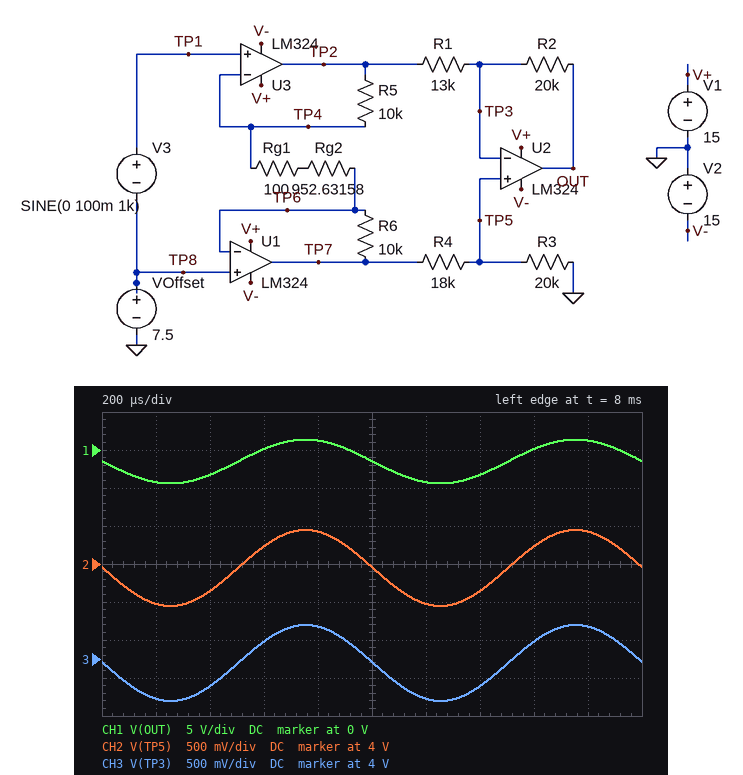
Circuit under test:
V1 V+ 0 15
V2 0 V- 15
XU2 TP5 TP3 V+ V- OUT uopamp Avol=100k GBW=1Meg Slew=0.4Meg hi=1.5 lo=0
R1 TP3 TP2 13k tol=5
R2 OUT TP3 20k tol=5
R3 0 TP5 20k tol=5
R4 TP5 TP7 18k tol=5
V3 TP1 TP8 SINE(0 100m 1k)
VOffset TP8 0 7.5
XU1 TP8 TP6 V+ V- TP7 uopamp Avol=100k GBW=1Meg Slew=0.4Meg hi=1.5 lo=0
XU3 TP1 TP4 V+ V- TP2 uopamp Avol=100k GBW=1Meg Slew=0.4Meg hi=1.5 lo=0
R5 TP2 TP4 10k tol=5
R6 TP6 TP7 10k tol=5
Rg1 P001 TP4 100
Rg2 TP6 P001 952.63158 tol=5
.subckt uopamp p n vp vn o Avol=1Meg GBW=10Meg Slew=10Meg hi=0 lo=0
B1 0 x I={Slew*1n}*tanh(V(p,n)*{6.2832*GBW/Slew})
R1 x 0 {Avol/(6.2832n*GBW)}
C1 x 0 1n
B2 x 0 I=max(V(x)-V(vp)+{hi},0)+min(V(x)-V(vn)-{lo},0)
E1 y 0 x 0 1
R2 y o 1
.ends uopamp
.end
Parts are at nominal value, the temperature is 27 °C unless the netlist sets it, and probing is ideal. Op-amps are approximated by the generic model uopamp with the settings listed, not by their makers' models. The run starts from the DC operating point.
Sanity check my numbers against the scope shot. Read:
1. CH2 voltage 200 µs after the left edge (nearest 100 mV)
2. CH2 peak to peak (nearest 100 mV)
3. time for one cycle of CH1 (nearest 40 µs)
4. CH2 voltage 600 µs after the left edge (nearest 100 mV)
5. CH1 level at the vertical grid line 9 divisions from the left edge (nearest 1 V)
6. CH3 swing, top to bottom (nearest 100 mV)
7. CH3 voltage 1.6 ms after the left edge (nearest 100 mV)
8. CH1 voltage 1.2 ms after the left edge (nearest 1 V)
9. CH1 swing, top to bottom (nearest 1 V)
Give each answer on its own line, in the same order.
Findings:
3.5 V
1.0 V
1.00 ms
4.2 V
1 V
1.0 V
4.2 V
-4 V
6 V
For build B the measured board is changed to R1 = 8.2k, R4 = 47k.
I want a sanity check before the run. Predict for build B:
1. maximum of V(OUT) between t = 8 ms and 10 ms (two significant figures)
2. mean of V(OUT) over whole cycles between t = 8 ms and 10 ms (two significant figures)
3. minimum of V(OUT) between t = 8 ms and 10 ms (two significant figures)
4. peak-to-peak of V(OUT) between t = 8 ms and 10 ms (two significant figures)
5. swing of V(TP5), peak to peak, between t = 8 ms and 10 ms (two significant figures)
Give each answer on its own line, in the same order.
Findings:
-7.1 V
-11 V
-14 V
7.1 V
570 mV
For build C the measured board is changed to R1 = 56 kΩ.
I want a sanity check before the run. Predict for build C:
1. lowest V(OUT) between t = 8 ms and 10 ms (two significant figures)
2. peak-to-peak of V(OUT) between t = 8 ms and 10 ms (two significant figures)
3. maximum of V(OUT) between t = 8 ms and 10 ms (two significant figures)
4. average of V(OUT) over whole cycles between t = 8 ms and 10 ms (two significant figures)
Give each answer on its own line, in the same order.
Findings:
1.6 V
2.1 V
3.7 V
2.7 V
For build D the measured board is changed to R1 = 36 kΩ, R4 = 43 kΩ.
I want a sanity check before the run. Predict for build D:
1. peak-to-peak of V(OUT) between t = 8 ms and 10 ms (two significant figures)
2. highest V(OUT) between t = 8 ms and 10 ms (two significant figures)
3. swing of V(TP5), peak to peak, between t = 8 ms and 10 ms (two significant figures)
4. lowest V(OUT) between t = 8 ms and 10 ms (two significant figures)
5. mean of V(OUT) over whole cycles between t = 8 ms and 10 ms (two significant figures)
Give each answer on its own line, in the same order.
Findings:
2.1 V
590 mV
600 mV
-1.5 V
-460 mV
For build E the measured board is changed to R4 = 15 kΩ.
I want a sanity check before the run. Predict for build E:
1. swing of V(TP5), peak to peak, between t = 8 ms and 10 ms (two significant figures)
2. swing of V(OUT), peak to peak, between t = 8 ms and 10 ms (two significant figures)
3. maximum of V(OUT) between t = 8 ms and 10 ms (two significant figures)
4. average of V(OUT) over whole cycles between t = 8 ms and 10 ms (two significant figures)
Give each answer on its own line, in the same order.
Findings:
1.1 V
6.0 V
2.3 V
-660 mV
